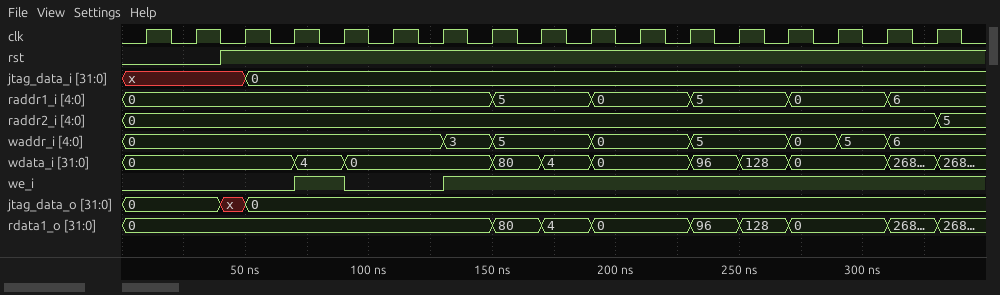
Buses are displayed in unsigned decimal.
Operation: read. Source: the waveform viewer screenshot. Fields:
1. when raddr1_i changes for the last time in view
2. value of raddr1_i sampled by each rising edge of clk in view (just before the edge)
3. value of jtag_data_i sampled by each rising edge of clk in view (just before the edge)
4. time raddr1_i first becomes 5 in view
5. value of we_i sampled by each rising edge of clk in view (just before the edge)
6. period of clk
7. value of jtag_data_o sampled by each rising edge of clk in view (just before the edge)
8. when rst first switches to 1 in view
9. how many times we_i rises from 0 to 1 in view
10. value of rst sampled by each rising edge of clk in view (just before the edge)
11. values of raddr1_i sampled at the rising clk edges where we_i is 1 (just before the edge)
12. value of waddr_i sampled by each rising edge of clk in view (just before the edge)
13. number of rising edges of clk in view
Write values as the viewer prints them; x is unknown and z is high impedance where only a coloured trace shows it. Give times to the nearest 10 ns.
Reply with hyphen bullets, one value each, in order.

- 310 ns
- 0, 0, 0, 0, 0, 0, 0, 0, 5, 5, 0, 0, 5, 5, 0, 0, 6
- x, x, x, 0, 0, 0, 0, 0, 0, 0, 0, 0, 0, 0, 0, 0, 0
- 150 ns
- 0 0 0 0 1 0 0 1 1 1 1 1 1 1 1 1 1
- 20 ns
- 0, 0, x, 0, 0, 0, 0, 0, 0, 0, 0, 0, 0, 0, 0, 0, 0
- 40 ns
- 2
- 0 0 1 1 1 1 1 1 1 1 1 1 1 1 1 1 1
- 0, 0, 5, 5, 0, 0, 5, 5, 0, 0, 6
- 0, 0, 0, 0, 0, 0, 0, 3, 5, 5, 0, 0, 5, 5, 0, 5, 6
- 17
